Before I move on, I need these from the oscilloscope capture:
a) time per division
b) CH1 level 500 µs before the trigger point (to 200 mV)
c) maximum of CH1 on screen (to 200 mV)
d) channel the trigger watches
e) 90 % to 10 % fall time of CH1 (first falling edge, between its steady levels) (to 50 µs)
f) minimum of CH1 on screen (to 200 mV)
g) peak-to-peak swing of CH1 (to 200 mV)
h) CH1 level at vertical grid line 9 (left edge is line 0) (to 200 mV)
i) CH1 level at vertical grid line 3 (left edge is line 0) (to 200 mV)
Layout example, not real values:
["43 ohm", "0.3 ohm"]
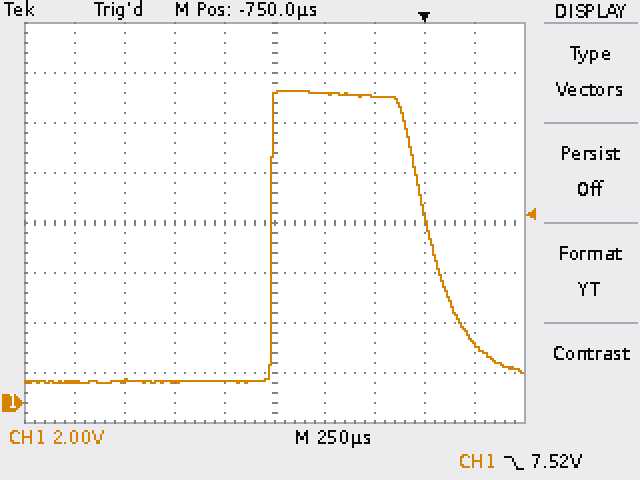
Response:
["250 µs", "12.4 V", "12.4 V", "CH1", "400 µs", "800 mV", "11.6 V", "2.4 V", "800 mV"]
